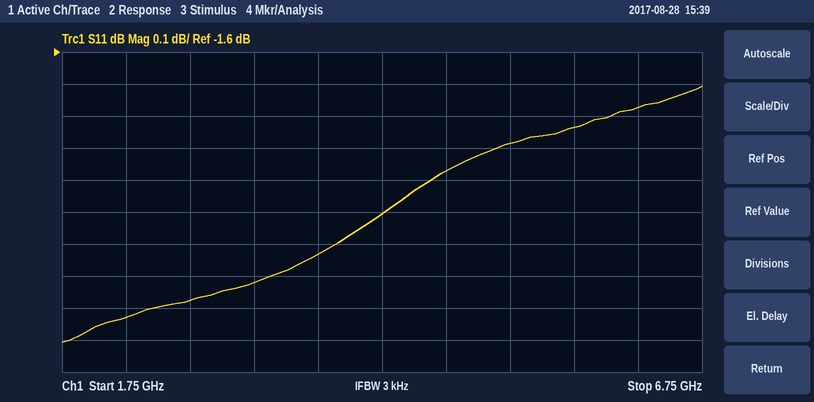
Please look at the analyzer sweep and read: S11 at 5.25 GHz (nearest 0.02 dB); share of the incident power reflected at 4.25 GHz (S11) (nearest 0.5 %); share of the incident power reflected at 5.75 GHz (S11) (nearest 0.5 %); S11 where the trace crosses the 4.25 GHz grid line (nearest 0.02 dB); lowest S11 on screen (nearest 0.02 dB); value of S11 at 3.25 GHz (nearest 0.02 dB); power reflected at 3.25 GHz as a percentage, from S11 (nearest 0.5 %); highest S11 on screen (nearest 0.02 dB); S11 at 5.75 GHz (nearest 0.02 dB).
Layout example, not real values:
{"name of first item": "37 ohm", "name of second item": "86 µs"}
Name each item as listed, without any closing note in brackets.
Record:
{"S11 at 5.25 GHz": "-1.88 dB", "share of the incident power reflected at 4.25 GHz (S11)": "61.5 %", "share of the incident power reflected at 5.75 GHz (S11)": "65.5 %", "S11 where the trace crosses the 4.25 GHz grid line": "-2.10 dB", "lowest S11 on screen": "-2.50 dB", "value of S11 at 3.25 GHz": "-2.32 dB", "power reflected at 3.25 GHz as a percentage, from S11": "58.5 %", "highest S11 on screen": "-1.70 dB", "S11 at 5.75 GHz": "-1.84 dB"}
